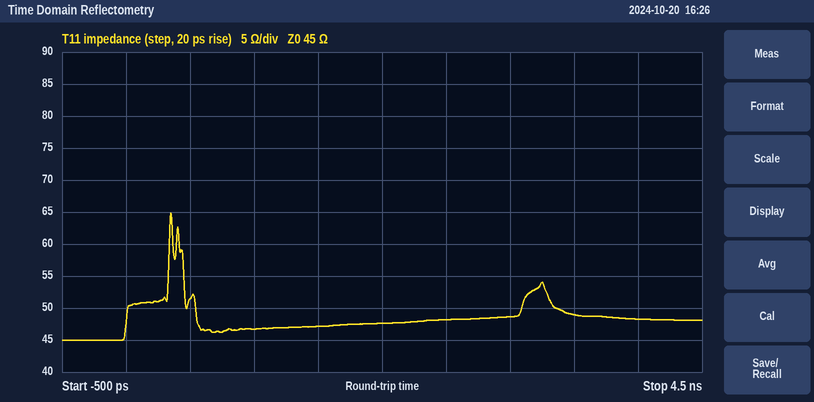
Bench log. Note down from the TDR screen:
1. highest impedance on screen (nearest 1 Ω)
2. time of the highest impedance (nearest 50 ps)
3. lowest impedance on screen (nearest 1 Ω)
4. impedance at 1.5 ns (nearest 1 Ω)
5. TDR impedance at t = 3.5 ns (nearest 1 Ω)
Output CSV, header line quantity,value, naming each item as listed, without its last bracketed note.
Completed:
quantity,value
highest impedance on screen,65 Ω
time of the highest impedance,350 ps
lowest impedance on screen,45 Ω
impedance at 1.5 ns,47 Ω
TDR impedance at t = 3.5 ns,49 Ω
